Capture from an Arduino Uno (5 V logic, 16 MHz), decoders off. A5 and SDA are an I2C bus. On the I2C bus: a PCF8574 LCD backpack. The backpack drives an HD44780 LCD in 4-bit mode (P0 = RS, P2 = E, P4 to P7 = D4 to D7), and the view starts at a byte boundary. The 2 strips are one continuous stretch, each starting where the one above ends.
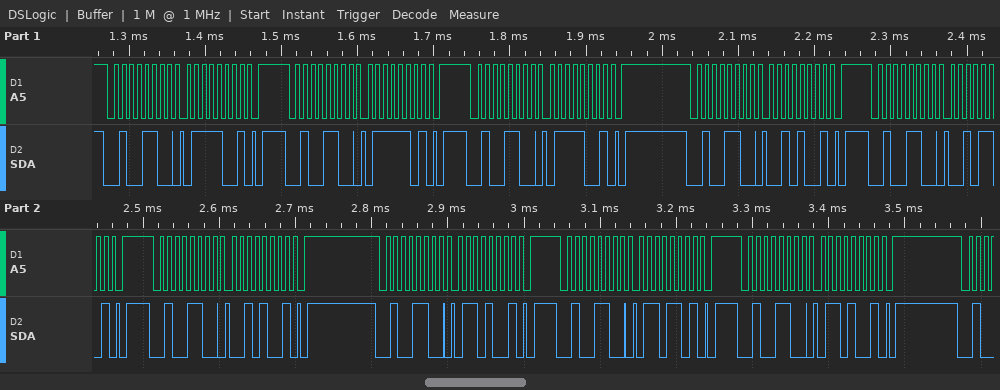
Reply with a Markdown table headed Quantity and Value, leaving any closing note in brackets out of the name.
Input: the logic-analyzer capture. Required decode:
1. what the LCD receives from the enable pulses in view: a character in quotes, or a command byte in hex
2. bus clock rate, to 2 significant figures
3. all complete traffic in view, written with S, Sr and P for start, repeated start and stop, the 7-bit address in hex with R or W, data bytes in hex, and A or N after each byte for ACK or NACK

| Quantity | Value |
|---|---|
| what the LCD receives from the enable pulses in view: a character in quotes, or a command byte in hex | 'r' |
| bus clock rate, to 2 significant figures | 100 kHz |
| all complete traffic in view, written with S, Sr and P for start, repeated start and stop, the 7-bit address in hex with R or W, data bytes in hex, and A or N after each byte for ACK or NACK | S 26W A 79 A P S 26W A 7D A P S 26W A 79 A P S 26W A 29 A P S 26W A 2D A P S 26W A 29 A P S 26W A 69 A P S 26W A 6D A P S 26W A 69 A P |
